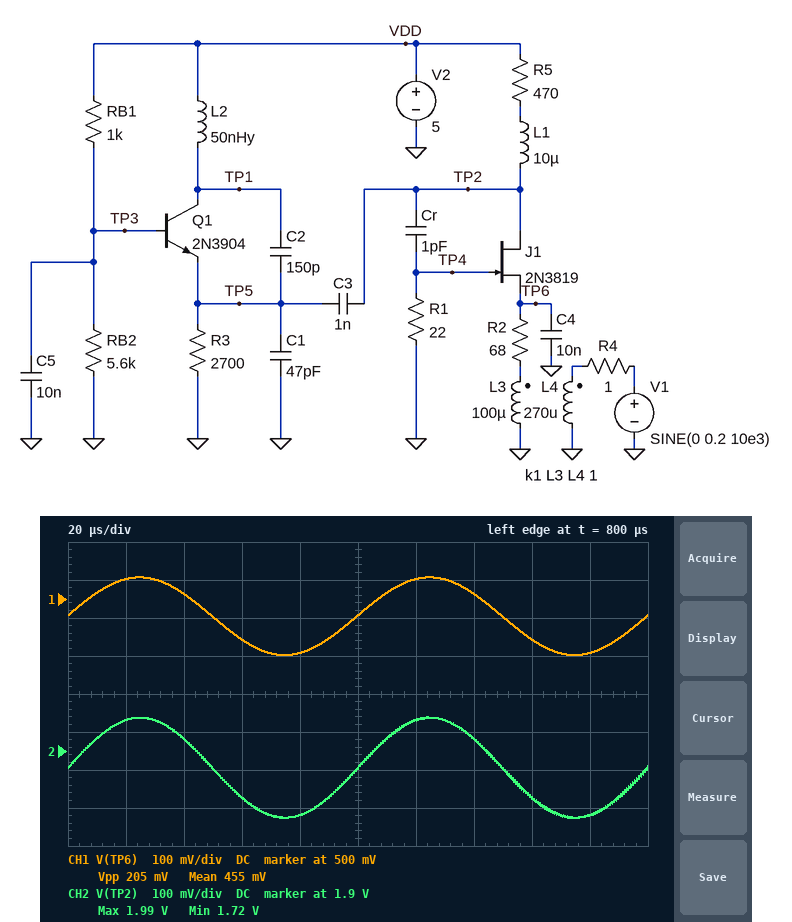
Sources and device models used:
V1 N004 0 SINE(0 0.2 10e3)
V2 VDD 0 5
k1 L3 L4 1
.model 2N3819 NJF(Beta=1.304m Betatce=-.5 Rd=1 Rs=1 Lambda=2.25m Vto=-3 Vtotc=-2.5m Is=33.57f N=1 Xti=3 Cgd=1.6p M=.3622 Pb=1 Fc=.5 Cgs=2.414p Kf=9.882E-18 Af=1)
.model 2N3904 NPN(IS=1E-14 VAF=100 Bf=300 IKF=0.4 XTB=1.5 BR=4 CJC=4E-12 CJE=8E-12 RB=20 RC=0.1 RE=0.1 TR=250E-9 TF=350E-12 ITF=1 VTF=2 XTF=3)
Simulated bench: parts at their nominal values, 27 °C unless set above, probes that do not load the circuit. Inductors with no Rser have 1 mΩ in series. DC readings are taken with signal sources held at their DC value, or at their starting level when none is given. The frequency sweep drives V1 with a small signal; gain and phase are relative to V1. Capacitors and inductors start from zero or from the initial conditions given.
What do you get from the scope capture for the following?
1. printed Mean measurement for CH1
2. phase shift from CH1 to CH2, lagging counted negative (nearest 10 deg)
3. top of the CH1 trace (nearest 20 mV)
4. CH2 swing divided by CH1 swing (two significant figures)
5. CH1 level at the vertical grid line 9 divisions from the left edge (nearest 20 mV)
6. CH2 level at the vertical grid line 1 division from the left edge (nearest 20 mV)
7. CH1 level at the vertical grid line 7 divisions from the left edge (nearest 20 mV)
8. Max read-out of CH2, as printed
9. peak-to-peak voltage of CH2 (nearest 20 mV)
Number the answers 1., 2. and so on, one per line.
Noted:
1. 455 mV
2. 0 deg
3. 560 mV
4. 1.3
5. 360 mV
6. 1.98 V
7. 520 mV
8. 1.99 V
9. 260 mV
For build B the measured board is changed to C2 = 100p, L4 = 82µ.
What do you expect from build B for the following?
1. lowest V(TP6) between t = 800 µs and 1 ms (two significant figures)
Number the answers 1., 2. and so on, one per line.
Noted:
1. 270 mV
